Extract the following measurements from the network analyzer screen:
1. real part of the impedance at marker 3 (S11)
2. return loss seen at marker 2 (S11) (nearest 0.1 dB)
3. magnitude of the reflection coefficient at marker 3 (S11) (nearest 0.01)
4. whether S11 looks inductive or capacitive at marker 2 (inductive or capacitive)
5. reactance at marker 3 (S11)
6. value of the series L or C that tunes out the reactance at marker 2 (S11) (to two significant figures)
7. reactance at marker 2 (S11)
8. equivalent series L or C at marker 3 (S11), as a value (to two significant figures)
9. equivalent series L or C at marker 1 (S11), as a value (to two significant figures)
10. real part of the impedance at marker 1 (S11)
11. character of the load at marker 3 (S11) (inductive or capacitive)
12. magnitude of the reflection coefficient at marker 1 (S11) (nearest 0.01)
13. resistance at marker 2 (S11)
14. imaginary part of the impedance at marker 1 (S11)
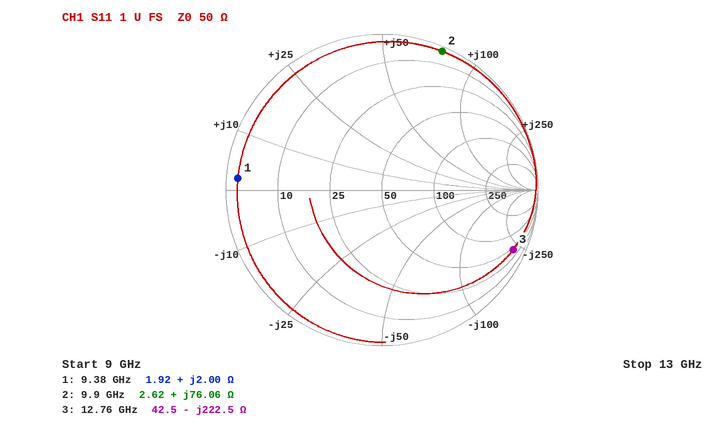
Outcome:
42.5 Ω
0.3 dB
0.92
inductive
-222.5 Ω
210 fF
+76.06 Ω
56 fF
34 pH
1.92 Ω
capacitive
0.93
2.62 Ω
+2.00 Ω
